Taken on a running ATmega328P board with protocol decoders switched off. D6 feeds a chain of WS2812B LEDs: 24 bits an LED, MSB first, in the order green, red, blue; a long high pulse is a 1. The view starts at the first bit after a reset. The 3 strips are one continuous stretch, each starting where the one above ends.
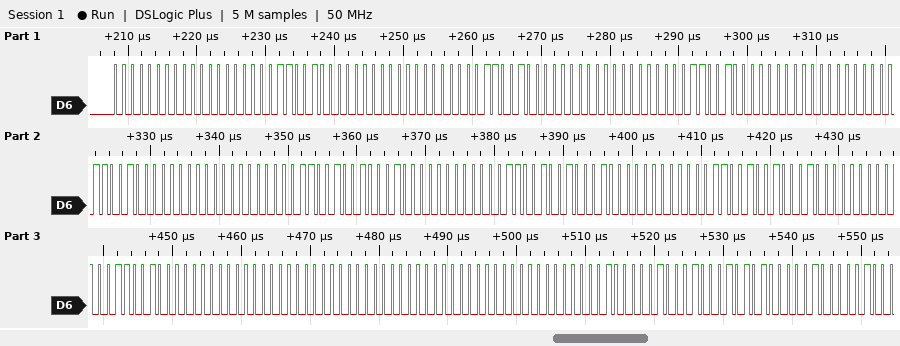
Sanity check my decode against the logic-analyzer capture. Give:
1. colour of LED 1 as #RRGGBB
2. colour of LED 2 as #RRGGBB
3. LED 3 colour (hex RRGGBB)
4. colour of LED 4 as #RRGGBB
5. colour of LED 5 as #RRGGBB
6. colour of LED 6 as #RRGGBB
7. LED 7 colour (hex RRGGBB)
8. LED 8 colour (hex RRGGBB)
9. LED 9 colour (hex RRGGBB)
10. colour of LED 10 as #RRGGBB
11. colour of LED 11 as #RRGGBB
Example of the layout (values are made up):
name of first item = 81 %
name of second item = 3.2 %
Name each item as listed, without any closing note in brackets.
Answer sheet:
colour of LED 1 as #RRGGBB = #000019
colour of LED 2 as #RRGGBB = #000019
LED 3 colour = #000019
colour of LED 4 as #RRGGBB = #000019
colour of LED 5 as #RRGGBB = #000019
colour of LED 6 as #RRGGBB = #002219
LED 7 colour = #002219
LED 8 colour = #002219
LED 9 colour = #000000
colour of LED 10 as #RRGGBB = #000000
colour of LED 11 as #RRGGBB = #22082A
